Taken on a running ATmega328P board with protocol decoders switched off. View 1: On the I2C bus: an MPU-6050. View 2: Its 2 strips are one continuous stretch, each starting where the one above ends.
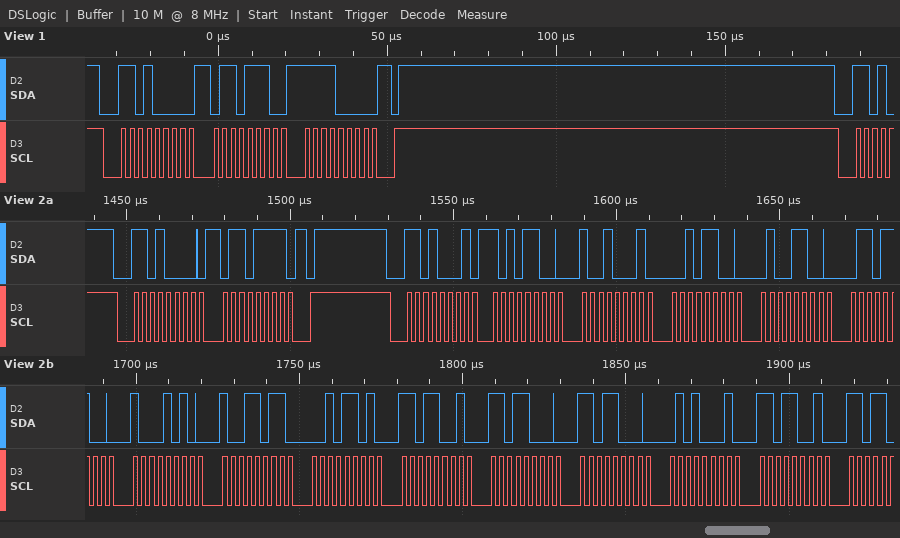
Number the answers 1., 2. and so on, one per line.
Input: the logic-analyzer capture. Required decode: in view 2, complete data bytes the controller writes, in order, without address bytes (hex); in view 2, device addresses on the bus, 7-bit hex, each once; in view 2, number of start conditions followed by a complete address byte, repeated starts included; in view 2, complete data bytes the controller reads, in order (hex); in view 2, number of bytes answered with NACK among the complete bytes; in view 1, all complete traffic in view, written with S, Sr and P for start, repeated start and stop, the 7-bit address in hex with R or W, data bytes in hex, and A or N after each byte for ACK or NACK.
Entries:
1. 6F
2. 0x68
3. 2
4. AC 91 2C 4C 6C 8A 9B 2D D9 D8 D8 51 D9
5. 0
6. S 68W A 6E A F0 A P
